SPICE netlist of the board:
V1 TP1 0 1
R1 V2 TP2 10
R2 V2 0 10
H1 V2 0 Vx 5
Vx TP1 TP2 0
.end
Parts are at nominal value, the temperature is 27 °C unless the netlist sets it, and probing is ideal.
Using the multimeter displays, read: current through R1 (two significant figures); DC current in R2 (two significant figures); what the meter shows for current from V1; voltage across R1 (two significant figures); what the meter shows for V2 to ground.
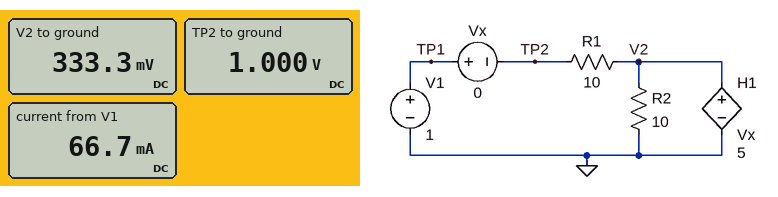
67 mA
33 mA
66.7 mA
670 mV
333.3 mV
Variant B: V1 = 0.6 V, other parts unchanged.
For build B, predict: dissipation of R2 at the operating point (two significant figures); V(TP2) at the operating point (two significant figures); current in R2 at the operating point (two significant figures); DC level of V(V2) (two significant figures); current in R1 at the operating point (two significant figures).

4.0 mW
600 mV
20 mA
200 mV
40 mA
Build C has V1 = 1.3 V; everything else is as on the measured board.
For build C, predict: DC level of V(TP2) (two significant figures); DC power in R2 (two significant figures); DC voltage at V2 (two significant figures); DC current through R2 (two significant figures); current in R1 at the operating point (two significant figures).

1.3 V
19 mW
430 mV
43 mA
87 mA
